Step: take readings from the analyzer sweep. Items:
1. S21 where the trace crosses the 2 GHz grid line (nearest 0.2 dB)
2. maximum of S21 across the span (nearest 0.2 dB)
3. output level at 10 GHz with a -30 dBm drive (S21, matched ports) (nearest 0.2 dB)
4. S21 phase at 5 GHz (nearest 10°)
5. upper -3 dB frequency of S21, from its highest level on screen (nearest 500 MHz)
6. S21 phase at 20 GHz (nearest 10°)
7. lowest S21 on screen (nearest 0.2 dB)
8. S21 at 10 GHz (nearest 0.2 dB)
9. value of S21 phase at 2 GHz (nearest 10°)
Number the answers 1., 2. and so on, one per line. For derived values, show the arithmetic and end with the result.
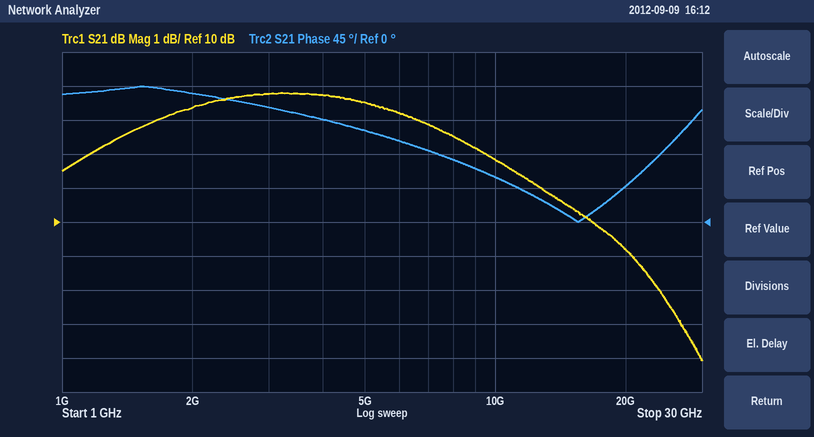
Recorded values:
1. 13.4 dB
2. 13.8 dB
3. -30 dBm + (11.8 dB) = -18.2 dBm
4. 120°
5. 13.5 GHz
6. 50°
7. 6.0 dB
8. 11.8 dB
9. 170°
